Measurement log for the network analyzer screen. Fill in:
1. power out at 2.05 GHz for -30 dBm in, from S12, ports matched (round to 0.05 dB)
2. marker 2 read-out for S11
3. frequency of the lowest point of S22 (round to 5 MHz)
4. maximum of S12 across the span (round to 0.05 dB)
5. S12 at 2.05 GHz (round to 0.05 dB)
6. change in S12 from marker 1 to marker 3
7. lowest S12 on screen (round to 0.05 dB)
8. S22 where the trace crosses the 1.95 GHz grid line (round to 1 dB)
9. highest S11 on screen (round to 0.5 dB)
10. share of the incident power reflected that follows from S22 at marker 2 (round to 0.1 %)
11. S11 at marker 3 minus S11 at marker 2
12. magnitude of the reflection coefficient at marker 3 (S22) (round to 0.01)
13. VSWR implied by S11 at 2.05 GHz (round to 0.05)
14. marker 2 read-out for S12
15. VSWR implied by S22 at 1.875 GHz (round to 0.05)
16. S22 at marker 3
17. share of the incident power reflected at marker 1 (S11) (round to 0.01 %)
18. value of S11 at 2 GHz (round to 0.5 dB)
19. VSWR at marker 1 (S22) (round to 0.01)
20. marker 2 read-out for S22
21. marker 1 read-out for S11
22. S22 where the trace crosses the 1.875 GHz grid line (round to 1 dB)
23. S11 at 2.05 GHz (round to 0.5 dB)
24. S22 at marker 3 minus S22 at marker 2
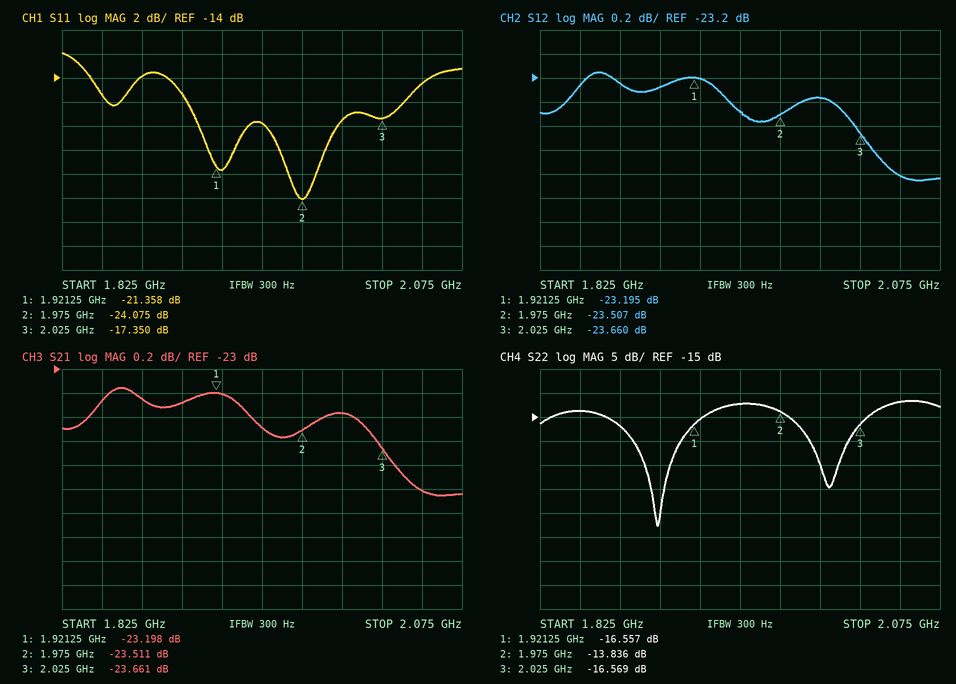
-54.00 dBm
-24.075 dB
1.900 GHz
-23.15 dB
-24.00 dB
-0.465 dB
-24.05 dB
-12 dB
-12.0 dB
4.1 %
6.725 dB
0.15
1.45
-23.507 dB
1.35
-16.569 dB
0.73 %
-17.5 dB
1.35
-13.836 dB
-21.358 dB
-17 dB
-14.5 dB
-2.733 dB
